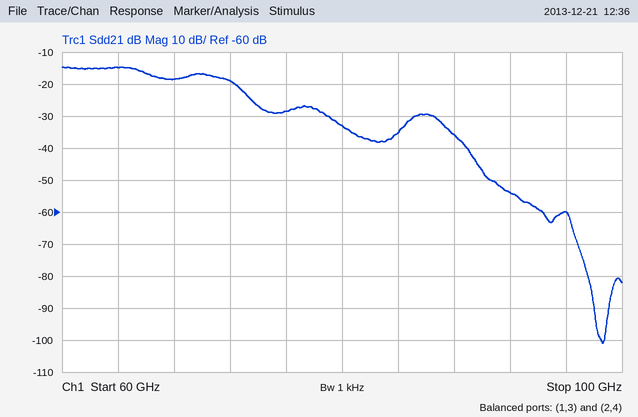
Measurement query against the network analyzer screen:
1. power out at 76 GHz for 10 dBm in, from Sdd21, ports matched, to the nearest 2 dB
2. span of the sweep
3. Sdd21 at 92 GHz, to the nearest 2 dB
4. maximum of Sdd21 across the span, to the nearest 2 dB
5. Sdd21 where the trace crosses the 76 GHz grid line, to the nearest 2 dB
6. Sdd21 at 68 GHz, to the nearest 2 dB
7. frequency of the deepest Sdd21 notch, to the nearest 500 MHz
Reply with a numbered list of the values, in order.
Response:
1. -18 dBm
2. 40 GHz
3. -54 dB
4. -14 dB
5. -28 dB
6. -18 dB
7. 98.5 GHz
